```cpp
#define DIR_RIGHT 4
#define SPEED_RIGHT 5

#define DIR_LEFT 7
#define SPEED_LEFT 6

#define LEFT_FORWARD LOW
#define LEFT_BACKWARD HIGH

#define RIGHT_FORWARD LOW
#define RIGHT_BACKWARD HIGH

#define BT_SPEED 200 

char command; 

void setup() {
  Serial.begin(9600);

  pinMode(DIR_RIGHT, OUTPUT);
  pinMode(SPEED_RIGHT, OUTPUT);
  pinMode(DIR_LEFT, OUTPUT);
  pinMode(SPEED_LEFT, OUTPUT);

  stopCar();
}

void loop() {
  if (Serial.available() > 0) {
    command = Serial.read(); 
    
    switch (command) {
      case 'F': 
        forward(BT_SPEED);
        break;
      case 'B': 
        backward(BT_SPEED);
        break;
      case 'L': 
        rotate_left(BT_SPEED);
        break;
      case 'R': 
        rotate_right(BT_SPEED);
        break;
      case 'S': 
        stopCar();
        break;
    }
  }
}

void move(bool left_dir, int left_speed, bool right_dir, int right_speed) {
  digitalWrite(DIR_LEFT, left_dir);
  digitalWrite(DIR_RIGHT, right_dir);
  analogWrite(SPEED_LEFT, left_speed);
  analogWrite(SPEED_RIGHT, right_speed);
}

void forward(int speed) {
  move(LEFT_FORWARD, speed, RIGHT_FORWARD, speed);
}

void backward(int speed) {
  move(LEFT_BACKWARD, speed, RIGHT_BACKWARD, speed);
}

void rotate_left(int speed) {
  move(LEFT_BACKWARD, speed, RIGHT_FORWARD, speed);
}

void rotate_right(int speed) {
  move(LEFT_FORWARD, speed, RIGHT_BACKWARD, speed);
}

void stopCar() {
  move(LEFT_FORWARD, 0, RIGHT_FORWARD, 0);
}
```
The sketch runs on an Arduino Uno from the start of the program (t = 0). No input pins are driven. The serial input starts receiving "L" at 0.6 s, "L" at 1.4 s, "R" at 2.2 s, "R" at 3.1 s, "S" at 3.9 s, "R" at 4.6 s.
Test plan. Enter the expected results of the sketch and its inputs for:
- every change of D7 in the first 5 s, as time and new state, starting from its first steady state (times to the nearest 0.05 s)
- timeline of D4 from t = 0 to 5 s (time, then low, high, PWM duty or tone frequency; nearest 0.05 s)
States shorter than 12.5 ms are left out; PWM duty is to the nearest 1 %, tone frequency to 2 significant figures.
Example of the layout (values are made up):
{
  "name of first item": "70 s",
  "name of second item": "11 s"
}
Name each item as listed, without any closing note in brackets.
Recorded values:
{
  "every change of D7 in the first 5 s, as time and new state, starting from its first steady state": "0 s low; 0.6 s high; 2.2 s low",
  "timeline of D4 from t = 0 to 5 s": "0 s low; 2.2 s high; 3.9 s low; 4.6 s high"
}
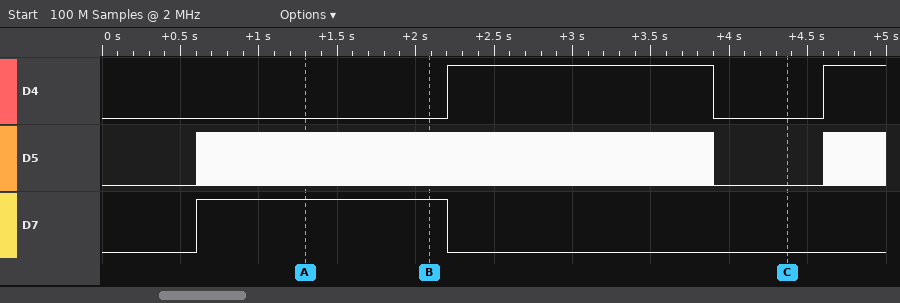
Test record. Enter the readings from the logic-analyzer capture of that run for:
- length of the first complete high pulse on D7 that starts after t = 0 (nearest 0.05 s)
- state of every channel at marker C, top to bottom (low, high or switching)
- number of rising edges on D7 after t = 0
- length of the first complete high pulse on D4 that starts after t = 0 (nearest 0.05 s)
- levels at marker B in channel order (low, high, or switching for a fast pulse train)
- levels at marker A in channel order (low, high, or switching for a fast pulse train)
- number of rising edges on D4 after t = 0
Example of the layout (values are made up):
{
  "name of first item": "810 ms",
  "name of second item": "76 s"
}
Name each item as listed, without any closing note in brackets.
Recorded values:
{
  "length of the first complete high pulse on D7 that starts after t = 0": "1.60 s",
  "state of every channel at marker C, top to bottom": "D4 low, D5 low, D7 low",
  "number of rising edges on D7 after t = 0": "1",
  "length of the first complete high pulse on D4 that starts after t = 0": "1.70 s",
  "levels at marker B in channel order": "D4 low, D5 switching, D7 high",
  "levels at marker A in channel order": "D4 low, D5 switching, D7 high",
  "number of rising edges on D4 after t = 0": "2"
}
